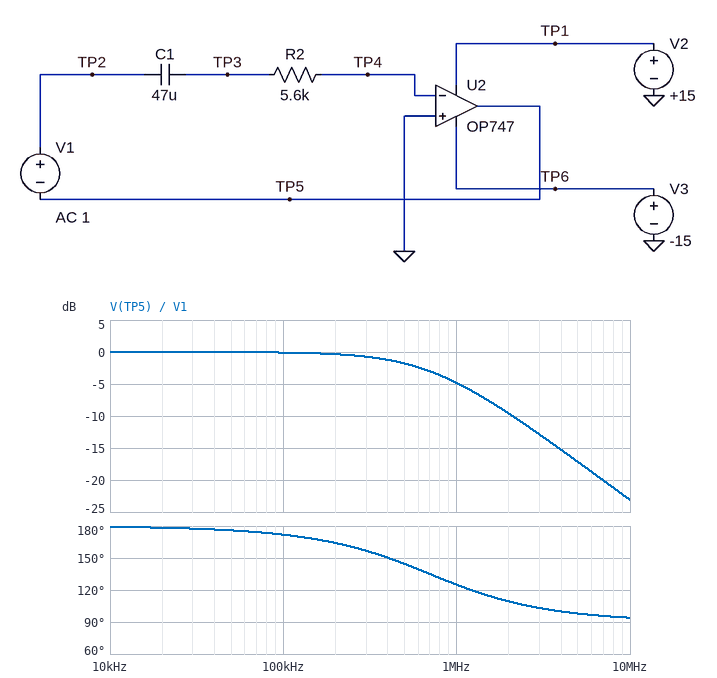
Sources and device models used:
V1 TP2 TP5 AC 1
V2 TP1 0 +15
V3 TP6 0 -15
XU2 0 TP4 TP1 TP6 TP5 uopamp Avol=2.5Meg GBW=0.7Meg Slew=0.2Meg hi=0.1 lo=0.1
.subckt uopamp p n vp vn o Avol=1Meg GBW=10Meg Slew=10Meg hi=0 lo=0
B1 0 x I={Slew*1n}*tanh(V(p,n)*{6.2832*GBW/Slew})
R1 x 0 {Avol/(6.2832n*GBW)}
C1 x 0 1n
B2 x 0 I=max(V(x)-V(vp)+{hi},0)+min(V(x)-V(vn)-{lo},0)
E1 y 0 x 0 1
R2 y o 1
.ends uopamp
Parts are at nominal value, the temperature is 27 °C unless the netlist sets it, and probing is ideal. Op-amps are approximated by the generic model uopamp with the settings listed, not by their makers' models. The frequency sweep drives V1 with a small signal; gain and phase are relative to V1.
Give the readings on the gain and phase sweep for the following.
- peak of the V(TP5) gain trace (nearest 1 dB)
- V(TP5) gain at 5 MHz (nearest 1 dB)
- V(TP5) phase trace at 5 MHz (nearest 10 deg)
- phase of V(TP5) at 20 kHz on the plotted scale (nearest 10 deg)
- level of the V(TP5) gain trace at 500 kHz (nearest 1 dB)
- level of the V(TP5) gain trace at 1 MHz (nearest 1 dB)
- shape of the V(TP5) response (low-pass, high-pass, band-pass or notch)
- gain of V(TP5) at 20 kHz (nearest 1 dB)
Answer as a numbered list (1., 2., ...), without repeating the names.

1. 0 dB
2. -17 dB
3. 100 deg
4. 180 deg
5. -2 dB
6. -5 dB
7. low-pass
8. 0 dB
